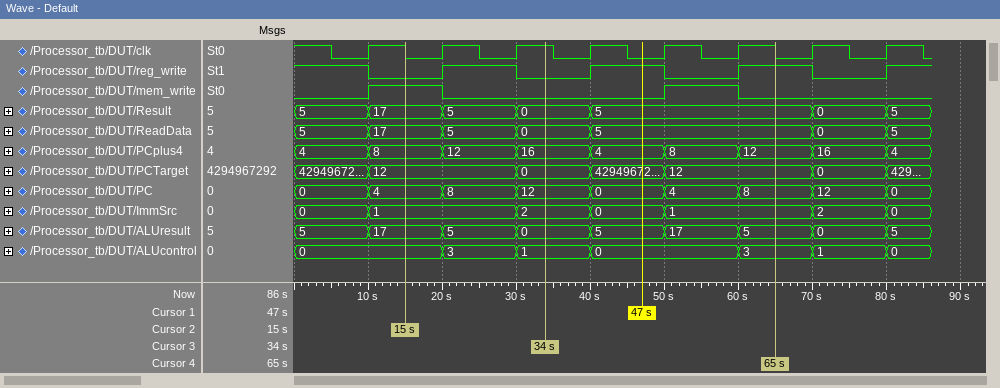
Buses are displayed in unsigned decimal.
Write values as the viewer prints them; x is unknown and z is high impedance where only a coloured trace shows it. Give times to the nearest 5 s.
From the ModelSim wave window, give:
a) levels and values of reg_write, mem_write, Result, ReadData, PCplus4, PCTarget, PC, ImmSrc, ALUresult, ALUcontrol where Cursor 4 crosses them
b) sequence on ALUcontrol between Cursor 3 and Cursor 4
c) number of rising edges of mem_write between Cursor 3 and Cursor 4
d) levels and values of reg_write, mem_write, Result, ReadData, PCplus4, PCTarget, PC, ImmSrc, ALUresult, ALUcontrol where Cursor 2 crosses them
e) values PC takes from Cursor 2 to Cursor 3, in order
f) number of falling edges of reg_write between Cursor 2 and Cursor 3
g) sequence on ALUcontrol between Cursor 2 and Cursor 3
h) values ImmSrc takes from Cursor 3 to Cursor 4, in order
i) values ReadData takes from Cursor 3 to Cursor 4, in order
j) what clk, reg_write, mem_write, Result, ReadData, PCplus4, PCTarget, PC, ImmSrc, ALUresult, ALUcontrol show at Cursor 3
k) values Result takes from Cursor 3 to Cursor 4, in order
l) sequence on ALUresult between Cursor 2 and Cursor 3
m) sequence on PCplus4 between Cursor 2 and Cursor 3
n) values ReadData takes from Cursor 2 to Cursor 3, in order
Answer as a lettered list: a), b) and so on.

a) reg_write=1, mem_write=0, Result=5, ReadData=5, PCplus4=12, PCTarget=12, PC=8, ImmSrc=1, ALUresult=5, ALUcontrol=3
b) 1, 0, 3
c) 1
d) reg_write=0, mem_write=1, Result=17, ReadData=17, PCplus4=8, PCTarget=12, PC=4, ImmSrc=1, ALUresult=17, ALUcontrol=0
e) 4, 8, 12
f) 1
g) 0, 3, 1
h) 2, 0, 1
i) 0, 5
j) clk=1, reg_write=0, mem_write=0, Result=0, ReadData=0, PCplus4=16, PCTarget=0, PC=12, ImmSrc=2, ALUresult=0, ALUcontrol=1
k) 0, 5
l) 17, 5, 0
m) 8, 12, 16
n) 17, 5, 0
